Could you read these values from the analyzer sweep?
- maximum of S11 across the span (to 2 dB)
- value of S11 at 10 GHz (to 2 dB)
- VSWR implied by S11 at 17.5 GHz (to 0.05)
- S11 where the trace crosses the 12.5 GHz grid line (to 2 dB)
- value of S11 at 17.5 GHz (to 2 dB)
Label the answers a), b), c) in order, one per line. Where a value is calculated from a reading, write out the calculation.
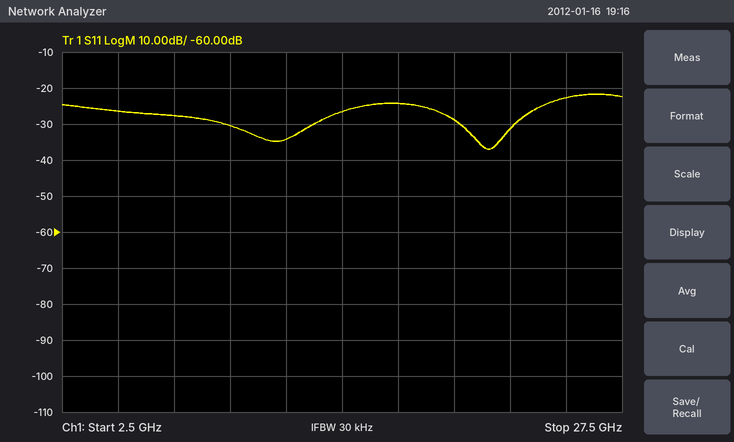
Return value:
a) -22 dB
b) -30 dB
c) |Γ| = 10^(-24/20) = 0.0631; VSWR = (1 + 0.0631)/(1 − 0.0631) ≈ 1.13, so 1.15 to the nearest 0.05
d) -34 dB
e) -24 dB
